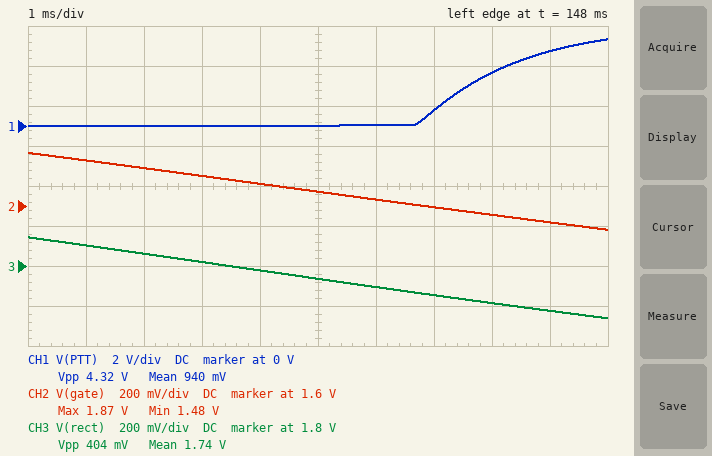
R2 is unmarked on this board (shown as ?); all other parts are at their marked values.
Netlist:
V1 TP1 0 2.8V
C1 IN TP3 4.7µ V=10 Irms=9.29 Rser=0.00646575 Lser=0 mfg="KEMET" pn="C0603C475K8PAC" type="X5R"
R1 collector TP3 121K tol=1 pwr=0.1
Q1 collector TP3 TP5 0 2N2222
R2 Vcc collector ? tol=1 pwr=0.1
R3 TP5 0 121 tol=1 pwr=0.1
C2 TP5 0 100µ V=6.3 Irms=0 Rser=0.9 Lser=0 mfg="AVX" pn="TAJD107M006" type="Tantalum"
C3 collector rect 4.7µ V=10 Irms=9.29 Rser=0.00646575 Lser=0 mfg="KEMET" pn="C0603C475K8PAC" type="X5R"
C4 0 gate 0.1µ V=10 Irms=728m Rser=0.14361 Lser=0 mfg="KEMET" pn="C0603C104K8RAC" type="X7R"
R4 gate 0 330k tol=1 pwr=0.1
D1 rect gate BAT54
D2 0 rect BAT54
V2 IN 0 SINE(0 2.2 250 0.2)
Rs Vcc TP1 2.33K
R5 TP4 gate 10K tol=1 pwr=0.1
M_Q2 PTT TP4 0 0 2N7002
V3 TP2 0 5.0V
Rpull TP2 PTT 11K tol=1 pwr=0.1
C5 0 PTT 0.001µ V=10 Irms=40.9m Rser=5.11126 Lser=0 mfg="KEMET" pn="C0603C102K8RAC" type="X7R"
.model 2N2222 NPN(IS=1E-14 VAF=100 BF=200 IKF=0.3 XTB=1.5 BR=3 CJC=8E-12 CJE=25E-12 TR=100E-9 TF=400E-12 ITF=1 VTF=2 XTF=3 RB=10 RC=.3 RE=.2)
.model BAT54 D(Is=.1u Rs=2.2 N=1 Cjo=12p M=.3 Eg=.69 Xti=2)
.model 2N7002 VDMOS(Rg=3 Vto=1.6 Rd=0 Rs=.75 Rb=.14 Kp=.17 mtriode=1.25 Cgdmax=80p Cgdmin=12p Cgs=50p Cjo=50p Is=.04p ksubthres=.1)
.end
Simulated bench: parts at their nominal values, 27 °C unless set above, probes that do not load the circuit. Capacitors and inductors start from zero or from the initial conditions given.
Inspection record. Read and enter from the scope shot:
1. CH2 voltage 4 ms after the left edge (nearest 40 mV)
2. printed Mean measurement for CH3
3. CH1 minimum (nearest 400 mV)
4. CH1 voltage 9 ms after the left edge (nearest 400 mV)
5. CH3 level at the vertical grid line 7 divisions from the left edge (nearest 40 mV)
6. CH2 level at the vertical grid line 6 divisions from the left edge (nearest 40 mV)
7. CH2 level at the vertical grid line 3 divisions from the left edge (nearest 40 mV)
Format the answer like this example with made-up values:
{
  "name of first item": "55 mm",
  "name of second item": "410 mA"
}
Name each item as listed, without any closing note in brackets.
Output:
{
  "CH2 voltage 4 ms after the left edge": "1.72 V",
  "printed Mean measurement for CH3": "1.74 V",
  "CH1 minimum": "0 V",
  "CH1 voltage 9 ms after the left edge": "3.6 V",
  "CH3 level at the vertical grid line 7 divisions from the left edge": "1.64 V",
  "CH2 level at the vertical grid line 6 divisions from the left edge": "1.64 V",
  "CH2 level at the vertical grid line 3 divisions from the left edge": "1.76 V"
}
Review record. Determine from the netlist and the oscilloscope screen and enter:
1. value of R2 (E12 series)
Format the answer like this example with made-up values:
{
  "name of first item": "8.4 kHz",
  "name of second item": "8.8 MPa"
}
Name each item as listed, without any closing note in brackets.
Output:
{
  "value of R2": "2.7 kΩ"
}
